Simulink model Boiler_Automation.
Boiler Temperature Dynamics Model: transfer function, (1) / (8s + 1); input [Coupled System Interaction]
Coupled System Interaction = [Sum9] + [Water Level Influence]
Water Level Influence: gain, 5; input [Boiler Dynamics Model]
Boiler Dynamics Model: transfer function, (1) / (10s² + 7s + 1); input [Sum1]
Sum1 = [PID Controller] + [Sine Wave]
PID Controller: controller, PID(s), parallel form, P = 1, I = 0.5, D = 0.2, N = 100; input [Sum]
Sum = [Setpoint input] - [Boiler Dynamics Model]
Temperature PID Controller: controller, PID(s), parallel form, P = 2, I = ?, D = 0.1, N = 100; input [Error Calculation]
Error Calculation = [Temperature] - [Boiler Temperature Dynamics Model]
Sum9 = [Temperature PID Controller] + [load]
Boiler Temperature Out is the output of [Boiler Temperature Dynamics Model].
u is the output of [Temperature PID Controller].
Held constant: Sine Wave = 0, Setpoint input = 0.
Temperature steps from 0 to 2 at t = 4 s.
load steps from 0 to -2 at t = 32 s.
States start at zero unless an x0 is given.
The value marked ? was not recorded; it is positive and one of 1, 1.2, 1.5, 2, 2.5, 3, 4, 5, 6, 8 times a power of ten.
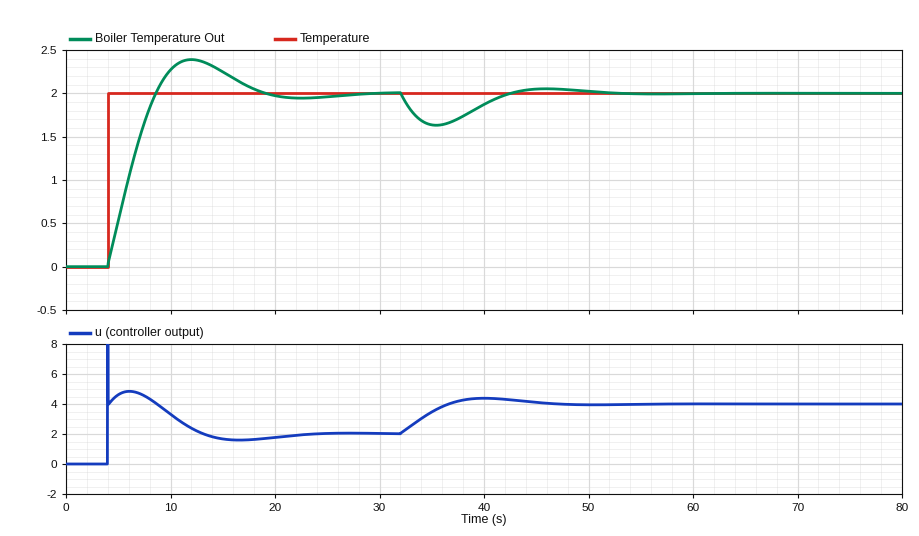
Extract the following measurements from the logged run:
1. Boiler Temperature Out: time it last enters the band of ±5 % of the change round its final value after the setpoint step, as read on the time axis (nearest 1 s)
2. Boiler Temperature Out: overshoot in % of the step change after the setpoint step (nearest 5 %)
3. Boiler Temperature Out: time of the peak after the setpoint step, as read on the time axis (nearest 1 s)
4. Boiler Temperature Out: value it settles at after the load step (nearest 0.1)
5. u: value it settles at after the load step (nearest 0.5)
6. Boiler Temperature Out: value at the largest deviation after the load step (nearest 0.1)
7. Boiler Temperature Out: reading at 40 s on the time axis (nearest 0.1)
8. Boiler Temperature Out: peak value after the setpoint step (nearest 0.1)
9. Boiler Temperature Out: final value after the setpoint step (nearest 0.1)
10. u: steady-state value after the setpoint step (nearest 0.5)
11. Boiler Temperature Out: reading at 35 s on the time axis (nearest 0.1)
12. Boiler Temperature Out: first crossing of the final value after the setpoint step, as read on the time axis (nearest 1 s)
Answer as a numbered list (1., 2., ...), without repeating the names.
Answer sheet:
1. 17 s
2. 20 %
3. 12 s
4. 2.0
5. 4.0
6. 1.6
7. 1.9
8. 2.4
9. 2.0
10. 2.0
11. 1.6
12. 9 s
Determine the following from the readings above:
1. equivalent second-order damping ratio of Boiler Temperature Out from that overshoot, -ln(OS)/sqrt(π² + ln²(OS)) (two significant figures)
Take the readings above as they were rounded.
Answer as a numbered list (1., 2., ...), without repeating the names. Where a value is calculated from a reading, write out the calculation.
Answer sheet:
1. ln(0.2) = -1.609; 1.609 / sqrt(9.870 + 2.590) = 0.46
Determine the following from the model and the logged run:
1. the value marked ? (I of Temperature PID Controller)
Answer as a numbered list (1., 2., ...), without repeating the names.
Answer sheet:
1. 1
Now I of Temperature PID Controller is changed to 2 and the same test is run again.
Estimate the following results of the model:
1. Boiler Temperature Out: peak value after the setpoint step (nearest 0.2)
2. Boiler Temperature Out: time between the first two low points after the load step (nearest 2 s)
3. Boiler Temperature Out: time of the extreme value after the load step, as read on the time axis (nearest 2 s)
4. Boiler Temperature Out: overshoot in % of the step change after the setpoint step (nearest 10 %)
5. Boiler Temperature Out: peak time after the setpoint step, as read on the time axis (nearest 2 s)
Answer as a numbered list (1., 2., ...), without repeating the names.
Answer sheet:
1. 2.6
2. 14 s
3. 34 s
4. 30 %
5. 10 s
